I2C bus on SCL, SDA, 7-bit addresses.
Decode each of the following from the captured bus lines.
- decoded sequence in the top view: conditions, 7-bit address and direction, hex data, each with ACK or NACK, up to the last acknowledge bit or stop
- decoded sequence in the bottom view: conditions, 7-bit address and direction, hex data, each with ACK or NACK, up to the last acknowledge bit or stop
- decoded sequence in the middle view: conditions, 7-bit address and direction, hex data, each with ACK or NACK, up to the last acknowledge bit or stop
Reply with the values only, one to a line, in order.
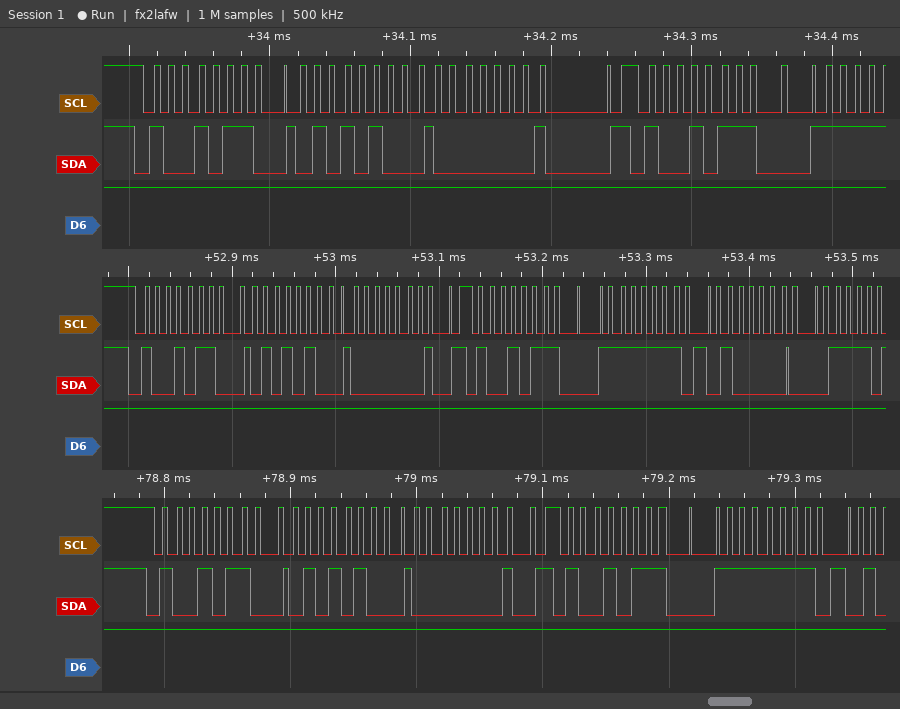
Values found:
start, address 4B write ACK, 54 ACK, 01 ACK, repeated start, address 4B read ACK
start, address 4B write ACK, 54 ACK, 01 ACK, repeated start, address 4B read ACK, FF ACK
start, address 4B write ACK, 54 ACK, 01 ACK, repeated start, address 4B read ACK, FF ACK, 20 ACK
